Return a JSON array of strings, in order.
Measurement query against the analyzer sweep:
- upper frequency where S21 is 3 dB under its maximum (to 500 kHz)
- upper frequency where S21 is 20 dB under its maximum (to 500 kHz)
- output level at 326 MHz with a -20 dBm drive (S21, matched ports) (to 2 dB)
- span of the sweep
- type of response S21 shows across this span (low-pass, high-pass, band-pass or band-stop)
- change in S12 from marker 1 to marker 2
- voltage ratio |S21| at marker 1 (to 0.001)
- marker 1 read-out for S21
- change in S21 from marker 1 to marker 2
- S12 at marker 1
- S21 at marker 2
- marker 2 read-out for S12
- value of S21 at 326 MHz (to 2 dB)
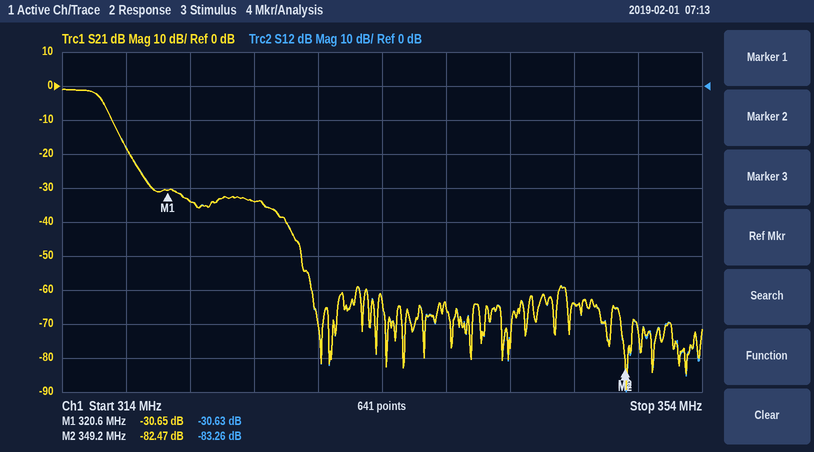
["316.5 MHz", "318.5 MHz", "-54 dBm", "40 MHz", "low-pass", "-52.63 dB", "0.029", "-30.65 dB", "-51.82 dB", "-30.63 dB", "-82.47 dB", "-83.26 dB", "-34 dB"]
